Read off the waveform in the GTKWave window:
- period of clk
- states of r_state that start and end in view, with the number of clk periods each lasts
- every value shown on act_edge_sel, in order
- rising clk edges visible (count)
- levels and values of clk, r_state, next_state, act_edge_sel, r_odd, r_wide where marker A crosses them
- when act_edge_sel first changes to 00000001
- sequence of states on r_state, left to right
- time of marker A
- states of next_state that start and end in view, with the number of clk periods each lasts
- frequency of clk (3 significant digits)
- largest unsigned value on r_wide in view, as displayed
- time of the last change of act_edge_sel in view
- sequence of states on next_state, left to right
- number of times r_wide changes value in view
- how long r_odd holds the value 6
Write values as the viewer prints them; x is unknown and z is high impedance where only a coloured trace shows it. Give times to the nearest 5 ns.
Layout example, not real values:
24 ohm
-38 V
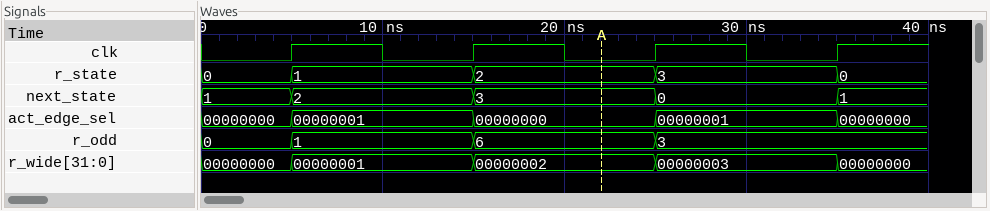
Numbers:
10 ns
1: 1, 2: 1, 3: 1
00000000, 00000001, 00000000, 00000001, 00000000
4
clk=0, r_state=2, next_state=3, act_edge_sel=00000000, r_odd=6, r_wide=00000002
5 ns
0, 1, 2, 3, 0
20 ns
2: 1, 3: 1, 0: 1
100 MHz
00000003
35 ns
1, 2, 3, 0, 1
4
10 ns
